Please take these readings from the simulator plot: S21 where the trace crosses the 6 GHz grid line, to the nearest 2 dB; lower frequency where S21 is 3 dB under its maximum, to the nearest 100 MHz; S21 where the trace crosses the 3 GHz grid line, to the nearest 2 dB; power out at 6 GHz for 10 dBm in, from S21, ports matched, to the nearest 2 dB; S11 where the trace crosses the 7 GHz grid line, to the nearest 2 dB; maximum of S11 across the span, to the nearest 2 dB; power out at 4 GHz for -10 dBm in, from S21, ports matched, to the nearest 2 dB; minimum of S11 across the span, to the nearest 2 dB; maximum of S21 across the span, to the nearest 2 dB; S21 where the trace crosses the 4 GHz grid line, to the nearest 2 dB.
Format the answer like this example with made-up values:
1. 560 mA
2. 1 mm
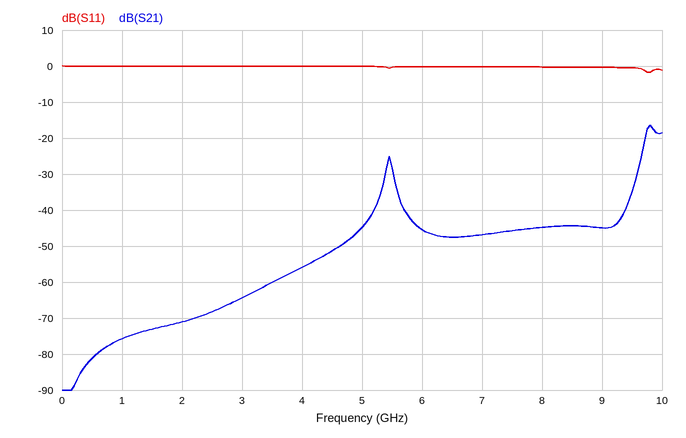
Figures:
1. -46 dB
2. 9.7 GHz
3. -64 dB
4. -36 dBm
5. 0 dB
6. 0 dB
7. -66 dBm
8. -2 dB
9. -16 dB
10. -56 dB
